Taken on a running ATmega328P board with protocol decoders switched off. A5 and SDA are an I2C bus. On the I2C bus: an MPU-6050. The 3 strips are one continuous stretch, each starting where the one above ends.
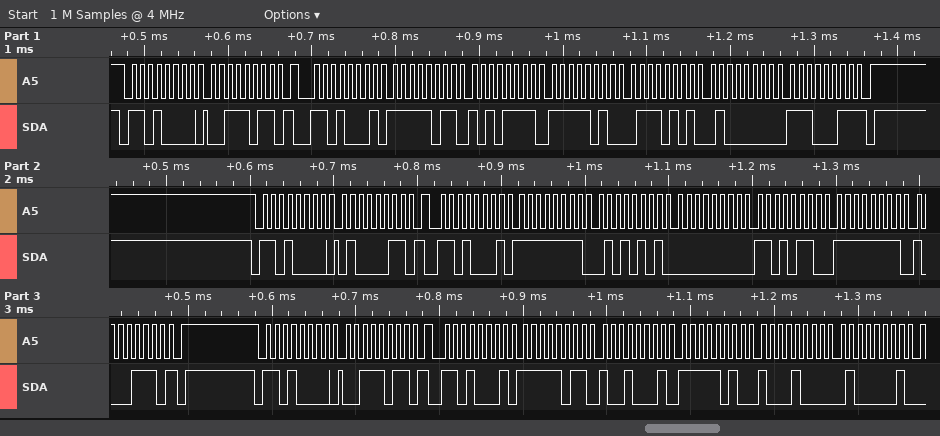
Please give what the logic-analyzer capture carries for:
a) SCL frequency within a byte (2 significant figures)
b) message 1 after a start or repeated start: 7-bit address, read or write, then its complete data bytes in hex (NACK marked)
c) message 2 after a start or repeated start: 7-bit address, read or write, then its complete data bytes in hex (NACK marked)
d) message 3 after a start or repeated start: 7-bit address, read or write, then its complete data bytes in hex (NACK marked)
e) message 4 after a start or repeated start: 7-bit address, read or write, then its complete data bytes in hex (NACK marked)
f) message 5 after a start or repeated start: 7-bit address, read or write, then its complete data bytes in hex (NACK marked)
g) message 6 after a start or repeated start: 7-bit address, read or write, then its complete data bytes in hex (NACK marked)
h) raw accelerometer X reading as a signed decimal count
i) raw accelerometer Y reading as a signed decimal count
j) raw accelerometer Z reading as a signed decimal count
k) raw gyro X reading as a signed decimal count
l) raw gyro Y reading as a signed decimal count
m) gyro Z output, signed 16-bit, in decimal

100 kHz
0x68 write: 3B
0x68 read: FB AF FA 75 40 E3 NACK
0x68 write: 43
0x68 read: FF 55 00 D6 FF 8E NACK
0x68 write: 3B
0x68 read: FB 91 FA 88 41
-1105
-1419
16611
-171
214
-114
